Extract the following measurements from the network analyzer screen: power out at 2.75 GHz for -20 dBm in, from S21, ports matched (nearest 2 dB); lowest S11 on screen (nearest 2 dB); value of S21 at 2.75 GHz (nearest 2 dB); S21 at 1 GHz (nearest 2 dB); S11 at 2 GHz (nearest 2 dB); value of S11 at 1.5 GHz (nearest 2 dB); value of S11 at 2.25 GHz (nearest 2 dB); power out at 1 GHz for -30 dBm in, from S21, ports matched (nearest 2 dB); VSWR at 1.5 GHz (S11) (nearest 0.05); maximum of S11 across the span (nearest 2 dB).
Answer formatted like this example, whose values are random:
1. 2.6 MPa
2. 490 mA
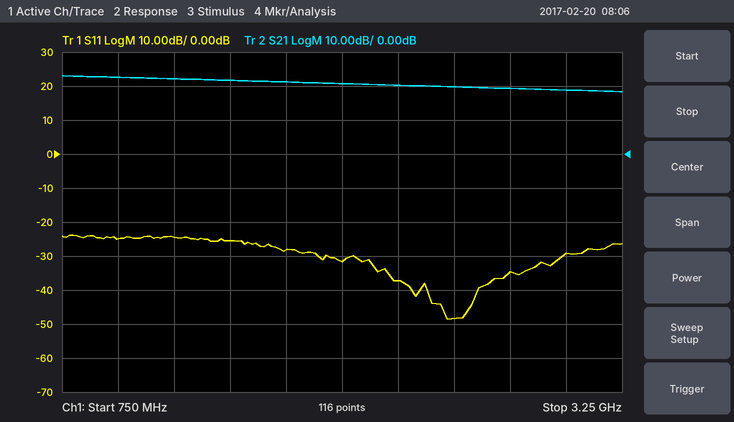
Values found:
1. 0 dBm
2. -48 dB
3. 20 dB
4. 22 dB
5. -32 dB
6. -26 dB
7. -38 dB
8. -8 dBm
9. 1.10
10. -24 dB
